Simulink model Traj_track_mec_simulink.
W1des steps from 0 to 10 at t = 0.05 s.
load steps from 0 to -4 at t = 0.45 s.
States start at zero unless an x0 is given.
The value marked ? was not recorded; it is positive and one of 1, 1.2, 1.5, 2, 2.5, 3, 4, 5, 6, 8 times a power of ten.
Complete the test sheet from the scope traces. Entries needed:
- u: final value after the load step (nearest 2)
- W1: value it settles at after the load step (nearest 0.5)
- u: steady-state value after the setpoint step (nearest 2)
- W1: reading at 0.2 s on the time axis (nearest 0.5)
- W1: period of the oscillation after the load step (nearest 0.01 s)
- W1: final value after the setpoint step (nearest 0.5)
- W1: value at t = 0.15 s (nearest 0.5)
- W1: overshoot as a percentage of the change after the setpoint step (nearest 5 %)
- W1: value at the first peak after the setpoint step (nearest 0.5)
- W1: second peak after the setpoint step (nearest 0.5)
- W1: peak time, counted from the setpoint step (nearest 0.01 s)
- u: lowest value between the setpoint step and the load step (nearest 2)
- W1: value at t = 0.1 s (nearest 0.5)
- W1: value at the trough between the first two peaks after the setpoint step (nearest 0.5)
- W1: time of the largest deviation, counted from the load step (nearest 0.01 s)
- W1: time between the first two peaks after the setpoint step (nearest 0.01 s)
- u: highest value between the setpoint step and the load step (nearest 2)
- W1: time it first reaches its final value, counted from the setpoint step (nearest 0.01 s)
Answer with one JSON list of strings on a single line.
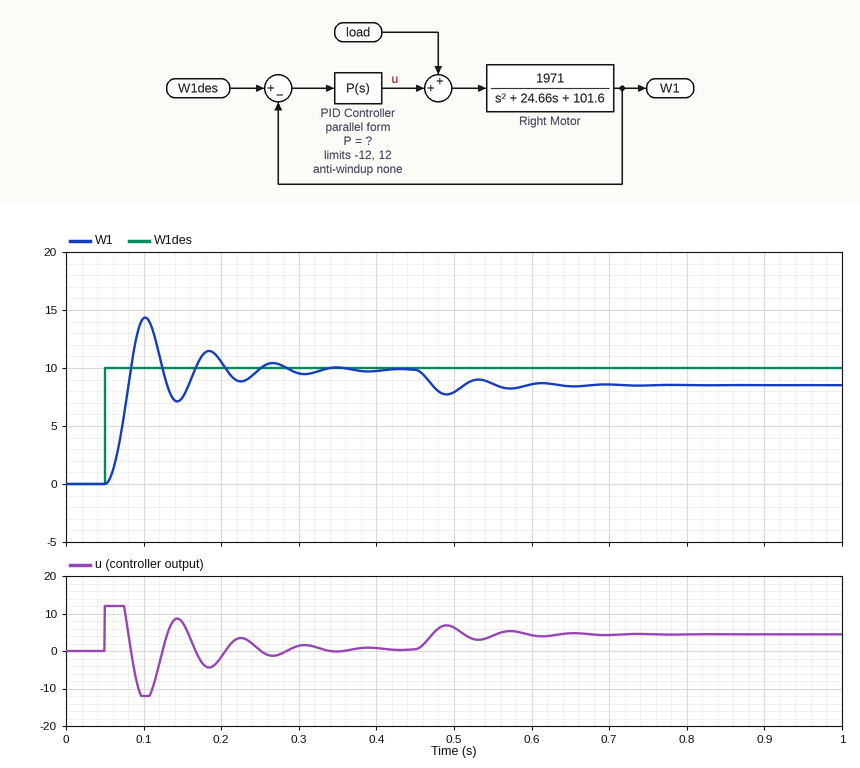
["4", "8.5", "0", "10.5", "0.08 s", "10.0", "7.5", "45 %", "14.5", "11.5", "0.05 s", "-12", "14.5", "7.0", "0.04 s", "0.08 s", "12", "0.03 s"]
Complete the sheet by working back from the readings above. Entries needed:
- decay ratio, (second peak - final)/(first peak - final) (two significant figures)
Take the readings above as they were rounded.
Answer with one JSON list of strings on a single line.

["0.33"]
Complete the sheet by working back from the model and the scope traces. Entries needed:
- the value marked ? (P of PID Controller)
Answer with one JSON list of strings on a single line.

["3"]
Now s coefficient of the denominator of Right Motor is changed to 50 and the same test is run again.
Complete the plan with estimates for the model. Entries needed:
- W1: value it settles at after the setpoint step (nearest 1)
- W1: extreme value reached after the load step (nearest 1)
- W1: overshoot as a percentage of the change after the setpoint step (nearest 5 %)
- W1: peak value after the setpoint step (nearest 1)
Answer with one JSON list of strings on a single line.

["10", "8", "25 %", "12"]
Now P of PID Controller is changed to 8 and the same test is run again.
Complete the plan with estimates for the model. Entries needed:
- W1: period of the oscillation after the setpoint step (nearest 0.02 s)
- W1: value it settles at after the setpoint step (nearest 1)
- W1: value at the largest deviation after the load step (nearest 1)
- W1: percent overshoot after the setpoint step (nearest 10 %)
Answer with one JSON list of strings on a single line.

["0.06 s", "10", "9", "40 %"]
